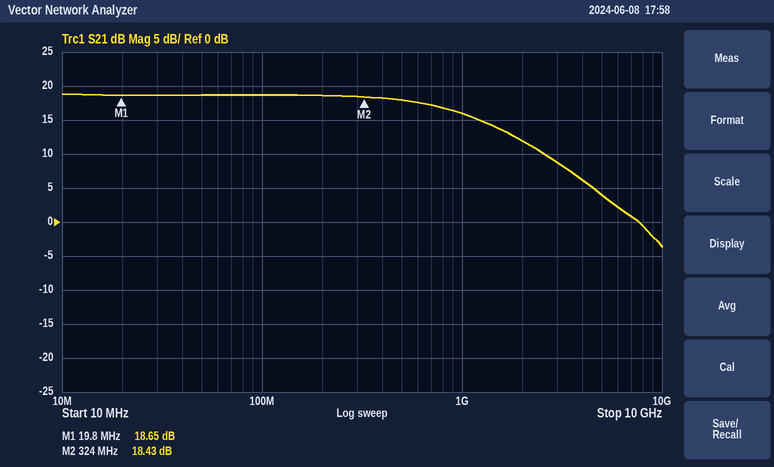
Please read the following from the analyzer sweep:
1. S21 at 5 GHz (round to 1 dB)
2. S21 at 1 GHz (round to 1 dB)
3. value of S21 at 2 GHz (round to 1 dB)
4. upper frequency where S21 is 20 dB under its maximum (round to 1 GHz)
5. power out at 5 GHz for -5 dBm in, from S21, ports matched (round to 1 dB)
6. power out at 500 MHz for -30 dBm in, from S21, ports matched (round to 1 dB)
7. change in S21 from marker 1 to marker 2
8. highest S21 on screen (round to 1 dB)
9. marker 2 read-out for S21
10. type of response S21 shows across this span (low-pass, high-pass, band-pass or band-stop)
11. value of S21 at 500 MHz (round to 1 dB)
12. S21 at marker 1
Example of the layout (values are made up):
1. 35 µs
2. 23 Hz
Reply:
1. 4 dB
2. 16 dB
3. 12 dB
4. 8 GHz
5. -1 dBm
6. -12 dBm
7. -0.22 dB
8. 19 dB
9. 18.43 dB
10. low-pass
11. 18 dB
12. 18.65 dB
